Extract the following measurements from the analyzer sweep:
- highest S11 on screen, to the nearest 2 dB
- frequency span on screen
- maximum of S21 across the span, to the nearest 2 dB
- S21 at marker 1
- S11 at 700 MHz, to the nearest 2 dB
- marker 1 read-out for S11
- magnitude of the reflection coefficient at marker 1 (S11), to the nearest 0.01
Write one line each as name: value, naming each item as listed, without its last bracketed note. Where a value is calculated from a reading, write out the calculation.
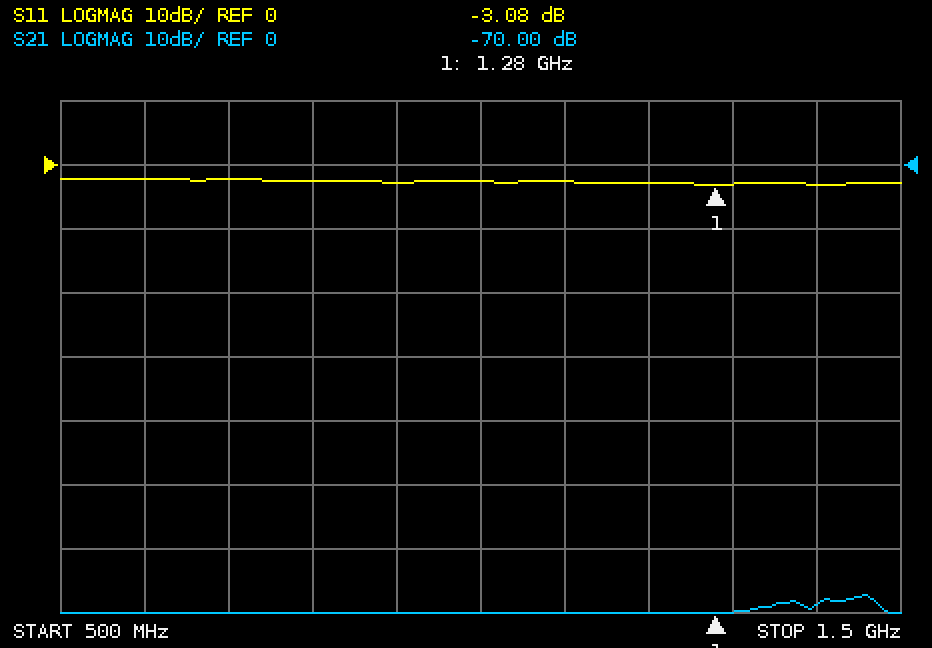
highest S11 on screen, to the nearest 2 dB: -2 dB
frequency span on screen: 1 GHz
maximum of S21 across the span, to the nearest 2 dB: -68 dB
S21 at marker 1: -70.00 dB
S11 at 700 MHz, to the nearest 2 dB: -2 dB
marker 1 read-out for S11: -3.08 dB
magnitude of the reflection coefficient at marker 1 (S11), to the nearest 0.01: 10^(-3.08/20) ≈ 0.70
